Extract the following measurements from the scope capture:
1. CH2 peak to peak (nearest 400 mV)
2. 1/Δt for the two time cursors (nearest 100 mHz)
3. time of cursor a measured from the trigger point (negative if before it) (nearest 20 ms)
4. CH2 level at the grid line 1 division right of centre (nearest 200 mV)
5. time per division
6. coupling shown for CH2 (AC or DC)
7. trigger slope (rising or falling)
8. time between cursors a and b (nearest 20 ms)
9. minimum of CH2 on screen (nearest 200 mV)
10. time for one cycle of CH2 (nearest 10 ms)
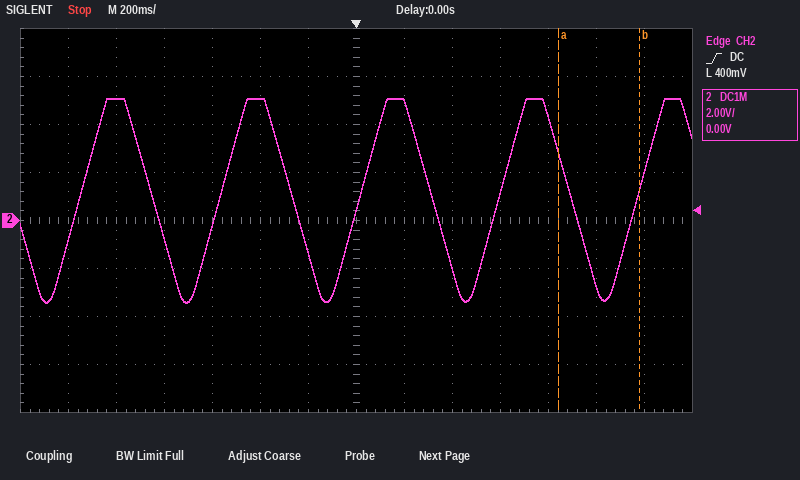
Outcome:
8.4 V
2.9 Hz
+840 ms
5.0 V
200 ms
DC
rising
340 ms
-3.4 V
580 ms
